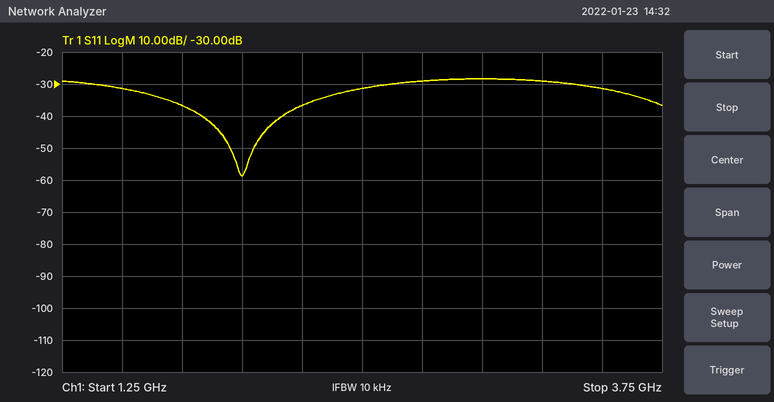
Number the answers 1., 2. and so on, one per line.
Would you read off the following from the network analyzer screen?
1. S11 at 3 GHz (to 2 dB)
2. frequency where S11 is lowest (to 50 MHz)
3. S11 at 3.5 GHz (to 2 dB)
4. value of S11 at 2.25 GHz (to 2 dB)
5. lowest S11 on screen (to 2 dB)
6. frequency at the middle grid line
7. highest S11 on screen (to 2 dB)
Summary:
1. -28 dB
2. 2.00 GHz
3. -32 dB
4. -36 dB
5. -58 dB
6. 2.5 GHz
7. -28 dB
